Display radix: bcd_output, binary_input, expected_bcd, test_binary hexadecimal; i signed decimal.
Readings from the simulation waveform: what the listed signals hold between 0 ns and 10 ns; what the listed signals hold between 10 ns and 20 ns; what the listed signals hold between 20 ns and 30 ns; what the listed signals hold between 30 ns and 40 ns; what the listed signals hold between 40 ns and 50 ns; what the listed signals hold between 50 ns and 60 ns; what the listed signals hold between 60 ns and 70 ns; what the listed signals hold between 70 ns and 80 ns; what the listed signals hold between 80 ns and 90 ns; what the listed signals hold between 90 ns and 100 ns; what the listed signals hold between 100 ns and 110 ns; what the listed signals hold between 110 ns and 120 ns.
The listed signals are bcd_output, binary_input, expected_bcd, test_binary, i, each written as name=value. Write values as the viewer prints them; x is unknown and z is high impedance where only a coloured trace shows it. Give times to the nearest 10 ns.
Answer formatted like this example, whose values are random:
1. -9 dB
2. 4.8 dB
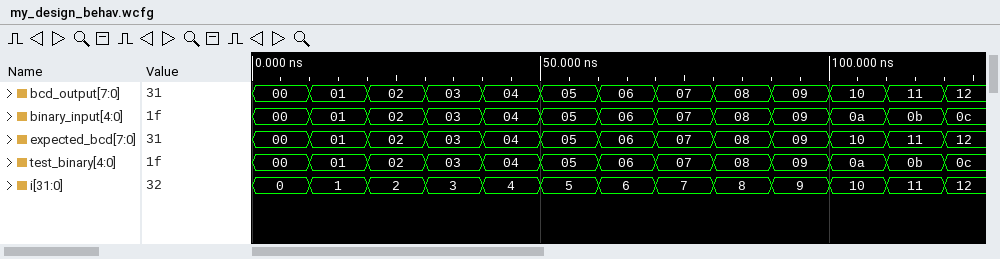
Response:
1. bcd_output=00, binary_input=00, expected_bcd=00, test_binary=00, i=0
2. bcd_output=01, binary_input=01, expected_bcd=01, test_binary=01, i=1
3. bcd_output=02, binary_input=02, expected_bcd=02, test_binary=02, i=2
4. bcd_output=03, binary_input=03, expected_bcd=03, test_binary=03, i=3
5. bcd_output=04, binary_input=04, expected_bcd=04, test_binary=04, i=4
6. bcd_output=05, binary_input=05, expected_bcd=05, test_binary=05, i=5
7. bcd_output=06, binary_input=06, expected_bcd=06, test_binary=06, i=6
8. bcd_output=07, binary_input=07, expected_bcd=07, test_binary=07, i=7
9. bcd_output=08, binary_input=08, expected_bcd=08, test_binary=08, i=8
10. bcd_output=09, binary_input=09, expected_bcd=09, test_binary=09, i=9
11. bcd_output=10, binary_input=0a, expected_bcd=10, test_binary=0a, i=10
12. bcd_output=11, binary_input=0b, expected_bcd=11, test_binary=0b, i=11
